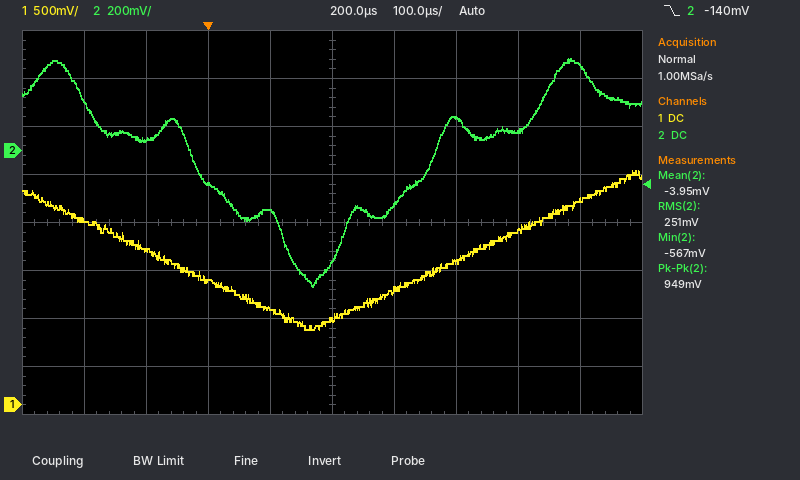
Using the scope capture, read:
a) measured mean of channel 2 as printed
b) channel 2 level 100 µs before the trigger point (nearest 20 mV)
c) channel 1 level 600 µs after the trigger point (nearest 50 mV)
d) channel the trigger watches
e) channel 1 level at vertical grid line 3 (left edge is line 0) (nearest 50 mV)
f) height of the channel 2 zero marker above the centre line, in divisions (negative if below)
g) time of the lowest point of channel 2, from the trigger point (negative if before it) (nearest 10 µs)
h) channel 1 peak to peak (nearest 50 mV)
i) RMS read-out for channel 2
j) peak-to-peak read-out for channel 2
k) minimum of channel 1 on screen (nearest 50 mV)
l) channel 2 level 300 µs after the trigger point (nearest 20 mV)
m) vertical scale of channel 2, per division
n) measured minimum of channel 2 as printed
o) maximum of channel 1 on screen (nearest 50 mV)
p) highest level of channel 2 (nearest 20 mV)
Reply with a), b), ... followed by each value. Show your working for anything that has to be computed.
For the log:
a) -3.95 mV
b) 40 mV
c) 2.15 V
d) channel 2
e) 1.30 V
f) +1.5 div
g) +170 µs
h) 2.45 V − (800 mV) = 1.65 V
i) 251 mV
j) 949 mV
k) 800 mV
l) -220 mV
m) 200 mV
n) -567 mV
o) 2.45 V
p) 380 mV
